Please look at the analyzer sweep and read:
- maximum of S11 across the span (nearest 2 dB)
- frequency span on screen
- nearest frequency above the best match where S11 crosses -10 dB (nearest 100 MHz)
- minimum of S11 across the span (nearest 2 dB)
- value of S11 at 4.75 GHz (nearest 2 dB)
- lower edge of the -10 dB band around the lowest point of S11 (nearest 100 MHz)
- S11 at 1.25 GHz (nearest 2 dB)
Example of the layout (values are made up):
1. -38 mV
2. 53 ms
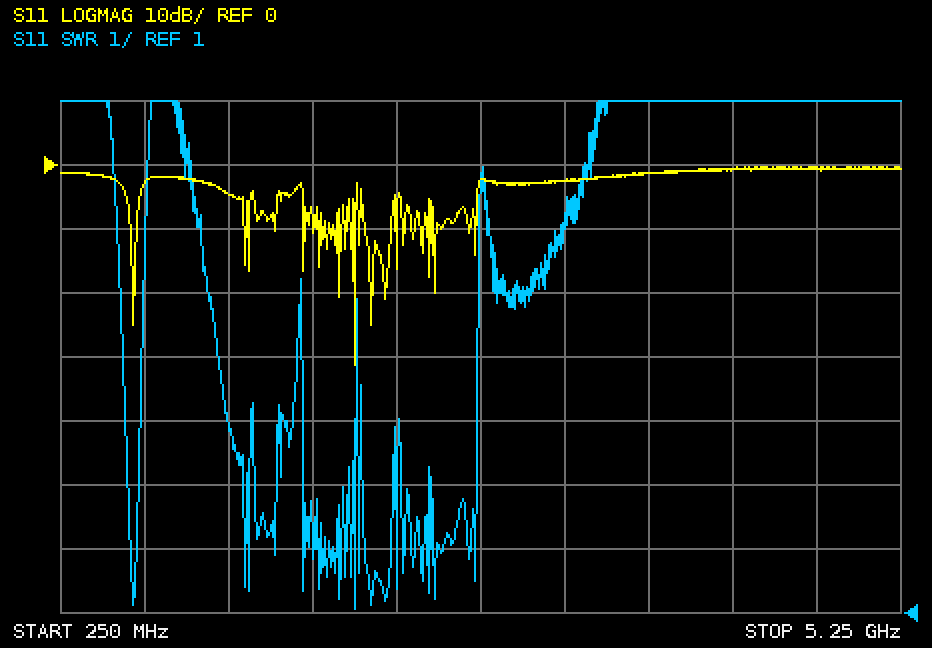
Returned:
1. 0 dB
2. 5 GHz
3. 2.0 GHz
4. -32 dB
5. 0 dB
6. 2.0 GHz
7. -4 dB
